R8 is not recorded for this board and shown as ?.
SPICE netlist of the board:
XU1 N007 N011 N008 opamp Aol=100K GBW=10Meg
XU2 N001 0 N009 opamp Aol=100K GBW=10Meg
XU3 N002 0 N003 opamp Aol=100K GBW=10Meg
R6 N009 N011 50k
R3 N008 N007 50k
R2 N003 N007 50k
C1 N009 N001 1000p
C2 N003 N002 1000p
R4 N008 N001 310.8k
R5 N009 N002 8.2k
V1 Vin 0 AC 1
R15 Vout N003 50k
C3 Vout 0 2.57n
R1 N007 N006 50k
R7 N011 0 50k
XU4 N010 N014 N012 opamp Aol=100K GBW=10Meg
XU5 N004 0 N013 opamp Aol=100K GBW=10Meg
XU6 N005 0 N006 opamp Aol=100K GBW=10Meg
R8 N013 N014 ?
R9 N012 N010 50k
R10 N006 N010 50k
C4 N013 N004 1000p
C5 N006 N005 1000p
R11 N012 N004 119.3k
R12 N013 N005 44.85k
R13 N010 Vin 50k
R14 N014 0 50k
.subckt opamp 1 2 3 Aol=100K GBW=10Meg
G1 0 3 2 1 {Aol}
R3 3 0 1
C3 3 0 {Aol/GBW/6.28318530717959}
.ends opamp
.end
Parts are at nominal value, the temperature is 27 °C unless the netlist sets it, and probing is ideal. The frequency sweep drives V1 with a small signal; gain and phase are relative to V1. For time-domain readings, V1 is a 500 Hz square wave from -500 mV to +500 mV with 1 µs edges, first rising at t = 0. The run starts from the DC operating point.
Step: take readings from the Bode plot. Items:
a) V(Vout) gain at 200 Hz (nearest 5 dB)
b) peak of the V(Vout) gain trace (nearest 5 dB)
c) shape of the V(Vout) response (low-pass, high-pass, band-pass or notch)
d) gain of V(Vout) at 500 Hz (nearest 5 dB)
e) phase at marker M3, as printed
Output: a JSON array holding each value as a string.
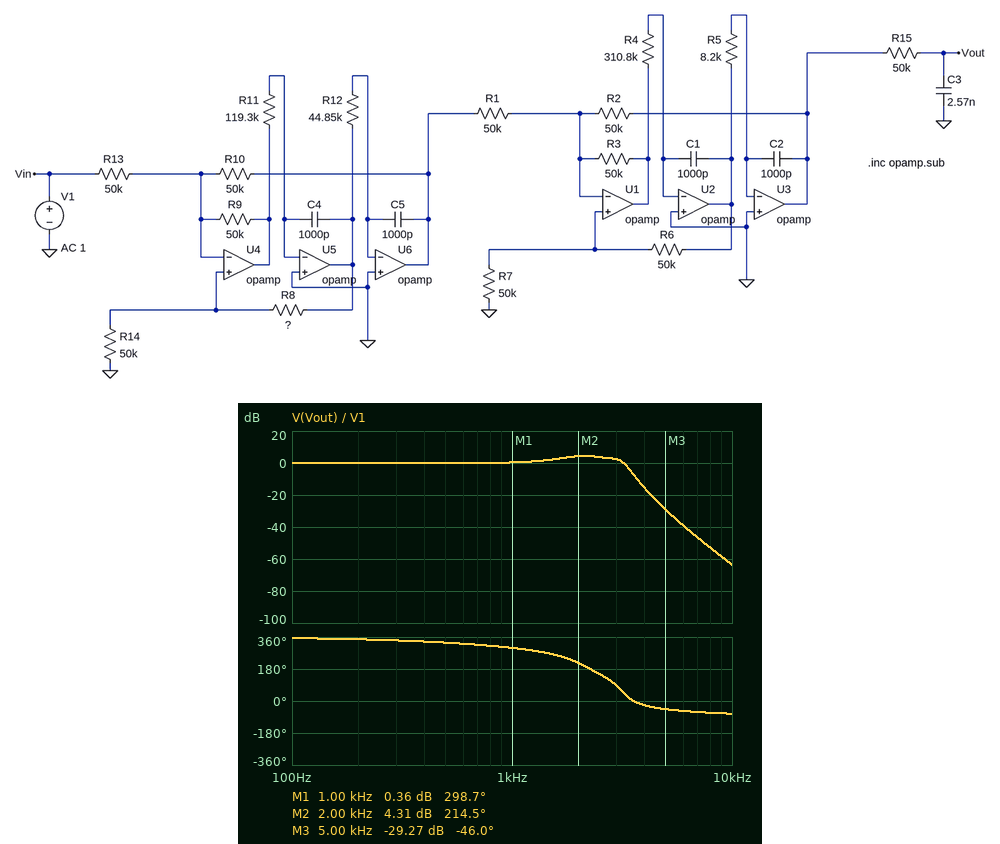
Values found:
["0 dB", "5 dB", "low-pass", "0 dB", "-46.0 deg"]
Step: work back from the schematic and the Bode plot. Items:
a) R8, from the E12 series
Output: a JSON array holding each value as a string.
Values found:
["120 kΩ"]
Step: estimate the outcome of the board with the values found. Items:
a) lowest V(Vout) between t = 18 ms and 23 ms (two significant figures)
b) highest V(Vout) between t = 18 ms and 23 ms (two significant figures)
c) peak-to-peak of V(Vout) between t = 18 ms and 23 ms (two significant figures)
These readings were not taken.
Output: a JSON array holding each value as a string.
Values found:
["-830 mV", "830 mV", "1.7 V"]
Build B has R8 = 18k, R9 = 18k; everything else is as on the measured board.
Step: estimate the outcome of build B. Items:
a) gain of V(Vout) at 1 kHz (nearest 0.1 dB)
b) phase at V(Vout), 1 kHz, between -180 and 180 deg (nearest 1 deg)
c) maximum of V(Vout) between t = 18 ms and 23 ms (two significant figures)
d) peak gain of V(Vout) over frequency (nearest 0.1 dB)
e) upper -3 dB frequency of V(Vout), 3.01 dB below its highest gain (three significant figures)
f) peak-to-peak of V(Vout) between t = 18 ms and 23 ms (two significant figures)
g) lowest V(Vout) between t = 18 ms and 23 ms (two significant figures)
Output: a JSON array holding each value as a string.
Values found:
["-1.9 dB", "-111 deg", "540 mV", "0 dB", "1.18 kHz", "1.1 V", "-540 mV"]
